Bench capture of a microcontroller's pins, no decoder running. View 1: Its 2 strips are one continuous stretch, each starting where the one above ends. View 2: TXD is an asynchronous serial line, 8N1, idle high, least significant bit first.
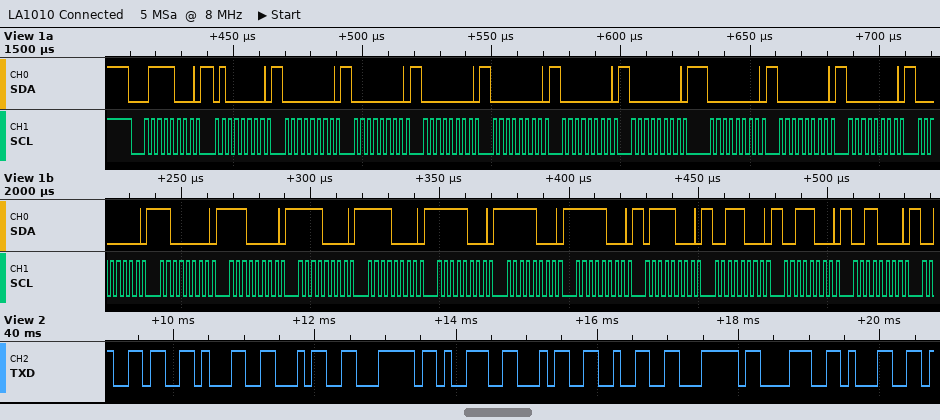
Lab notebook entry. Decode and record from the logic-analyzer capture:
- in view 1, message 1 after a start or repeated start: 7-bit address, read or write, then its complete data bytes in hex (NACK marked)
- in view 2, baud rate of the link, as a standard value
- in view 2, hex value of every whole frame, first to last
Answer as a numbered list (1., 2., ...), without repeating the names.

1. 0x3C write: 40 00 00 00 00 00 00 00 00 00 00 C0 E0 F0 F0 F8 F8 F8 78 38 38 30
2. 9600 baud
3. 0x36 0x31 0x34 0x7C 0x39 0x34 0x32 0x7C 0x38 0x31
